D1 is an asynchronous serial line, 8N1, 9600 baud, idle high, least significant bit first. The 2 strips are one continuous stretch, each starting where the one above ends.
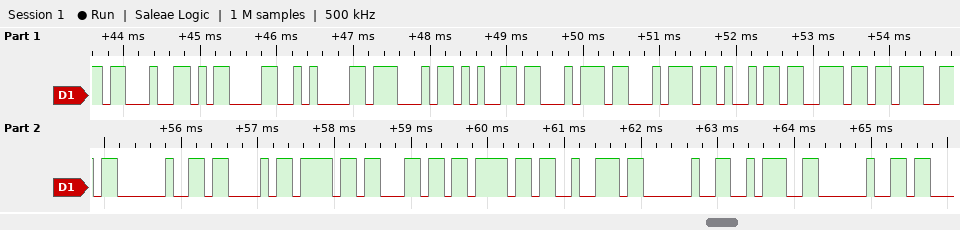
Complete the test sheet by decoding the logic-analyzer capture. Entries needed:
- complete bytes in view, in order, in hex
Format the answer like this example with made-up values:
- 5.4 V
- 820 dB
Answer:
- 23 0D 0A 47 65 74 74 69 6E 67 20 43 6F 6C 6F 72 20 3A 20
